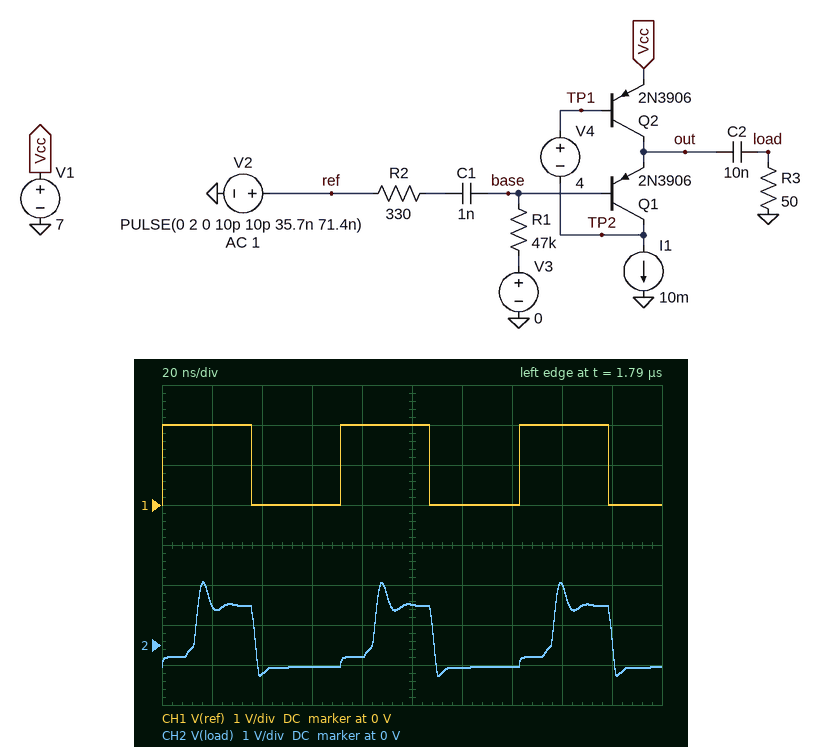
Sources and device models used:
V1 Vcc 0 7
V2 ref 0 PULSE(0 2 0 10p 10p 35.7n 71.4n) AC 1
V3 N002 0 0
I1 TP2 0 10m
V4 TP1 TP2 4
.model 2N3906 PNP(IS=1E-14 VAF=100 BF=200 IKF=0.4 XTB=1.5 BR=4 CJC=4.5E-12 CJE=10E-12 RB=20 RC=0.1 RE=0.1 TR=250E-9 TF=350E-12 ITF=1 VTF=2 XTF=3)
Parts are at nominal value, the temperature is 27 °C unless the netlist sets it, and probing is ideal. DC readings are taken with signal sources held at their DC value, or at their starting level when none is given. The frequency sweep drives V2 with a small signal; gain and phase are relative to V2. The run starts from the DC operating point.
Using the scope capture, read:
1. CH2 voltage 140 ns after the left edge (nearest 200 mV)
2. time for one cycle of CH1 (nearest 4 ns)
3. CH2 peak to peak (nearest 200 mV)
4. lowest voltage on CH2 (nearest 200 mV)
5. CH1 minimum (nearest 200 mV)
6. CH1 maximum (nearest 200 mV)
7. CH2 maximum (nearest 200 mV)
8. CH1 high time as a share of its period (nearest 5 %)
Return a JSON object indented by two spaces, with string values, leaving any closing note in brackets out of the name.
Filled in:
{
  "CH2 voltage 140 ns after the left edge": "-600 mV",
  "time for one cycle of CH1": "72 ns",
  "CH2 peak to peak": "2.4 V",
  "lowest voltage on CH2": "-800 mV",
  "CH1 minimum": "0 V",
  "CH1 maximum": "2.0 V",
  "CH2 maximum": "1.6 V",
  "CH1 high time as a share of its period": "50 %"
}
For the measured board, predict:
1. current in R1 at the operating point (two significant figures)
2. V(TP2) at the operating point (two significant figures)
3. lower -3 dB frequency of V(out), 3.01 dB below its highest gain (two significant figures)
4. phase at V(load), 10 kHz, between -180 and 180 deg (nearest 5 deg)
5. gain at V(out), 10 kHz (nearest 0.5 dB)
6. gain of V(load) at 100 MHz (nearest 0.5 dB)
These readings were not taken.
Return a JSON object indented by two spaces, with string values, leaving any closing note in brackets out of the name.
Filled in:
{
  "current in R1 at the operating point": "51 µA",
  "V(TP2) at the operating point": "2.3 V",
  "lower -3 dB frequency of V(out), 3.01 dB below its highest gain": "3.9 kHz",
  "phase at V(load), 10 kHz, between -180 and 180 deg": "105 deg",
  "gain at V(out), 10 kHz": "-0.5 dB",
  "gain of V(load) at 100 MHz": "-2.0 dB"
}
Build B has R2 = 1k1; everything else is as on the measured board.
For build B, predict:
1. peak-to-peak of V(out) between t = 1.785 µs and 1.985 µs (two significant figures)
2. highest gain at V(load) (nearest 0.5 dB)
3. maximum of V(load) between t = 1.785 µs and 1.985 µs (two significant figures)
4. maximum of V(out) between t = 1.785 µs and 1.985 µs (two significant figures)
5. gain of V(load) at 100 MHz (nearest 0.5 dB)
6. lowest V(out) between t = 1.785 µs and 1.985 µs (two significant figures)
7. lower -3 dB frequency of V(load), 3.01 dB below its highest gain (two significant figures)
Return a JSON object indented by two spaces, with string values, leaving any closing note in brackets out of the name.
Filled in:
{
  "peak-to-peak of V(out) between t = 1.785 µs and 1.985 µs": "1.7 V",
  "highest gain at V(load)": "-0.5 dB",
  "maximum of V(load) between t = 1.785 µs and 1.985 µs": "1.1 V",
  "maximum of V(out) between t = 1.785 µs and 1.985 µs": "5.1 V",
  "gain of V(load) at 100 MHz": "-13.0 dB",
  "lowest V(out) between t = 1.785 µs and 1.985 µs": "3.5 V",
  "lower -3 dB frequency of V(load), 3.01 dB below its highest gain": "310 kHz"
}
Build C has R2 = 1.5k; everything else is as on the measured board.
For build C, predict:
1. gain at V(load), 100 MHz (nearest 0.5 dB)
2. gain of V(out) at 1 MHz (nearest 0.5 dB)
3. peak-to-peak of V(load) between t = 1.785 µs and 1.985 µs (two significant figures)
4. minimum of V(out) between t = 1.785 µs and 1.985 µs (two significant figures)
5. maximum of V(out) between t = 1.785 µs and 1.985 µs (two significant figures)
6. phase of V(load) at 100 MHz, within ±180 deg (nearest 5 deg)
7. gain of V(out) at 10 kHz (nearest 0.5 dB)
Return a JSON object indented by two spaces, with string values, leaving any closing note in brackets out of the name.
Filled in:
{
  "gain at V(load), 100 MHz": "-16.0 dB",
  "gain of V(out) at 1 MHz": "-0.5 dB",
  "peak-to-peak of V(load) between t = 1.785 µs and 1.985 µs": "1.6 V",
  "minimum of V(out) between t = 1.785 µs and 1.985 µs": "3.5 V",
  "maximum of V(out) between t = 1.785 µs and 1.985 µs": "5.0 V",
  "phase of V(load) at 100 MHz, within ±180 deg": "-120 deg",
  "gain of V(out) at 10 kHz": "-1.0 dB"
}
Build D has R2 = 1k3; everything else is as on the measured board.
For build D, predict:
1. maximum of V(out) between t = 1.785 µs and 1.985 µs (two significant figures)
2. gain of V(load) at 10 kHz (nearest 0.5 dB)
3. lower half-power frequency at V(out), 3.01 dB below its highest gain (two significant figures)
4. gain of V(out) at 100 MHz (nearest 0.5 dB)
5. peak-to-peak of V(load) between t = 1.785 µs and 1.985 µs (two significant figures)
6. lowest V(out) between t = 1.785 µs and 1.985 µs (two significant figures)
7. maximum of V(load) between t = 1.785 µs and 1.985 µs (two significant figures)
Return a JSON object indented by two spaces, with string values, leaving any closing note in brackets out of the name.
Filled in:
{
  "maximum of V(out) between t = 1.785 µs and 1.985 µs": "5.1 V",
  "gain of V(load) at 10 kHz": "-31.0 dB",
  "lower half-power frequency at V(out), 3.01 dB below its highest gain": "3.4 kHz",
  "gain of V(out) at 100 MHz": "-14.5 dB",
  "peak-to-peak of V(load) between t = 1.785 µs and 1.985 µs": "1.6 V",
  "lowest V(out) between t = 1.785 µs and 1.985 µs": "3.5 V",
  "maximum of V(load) between t = 1.785 µs and 1.985 µs": "1.1 V"
}
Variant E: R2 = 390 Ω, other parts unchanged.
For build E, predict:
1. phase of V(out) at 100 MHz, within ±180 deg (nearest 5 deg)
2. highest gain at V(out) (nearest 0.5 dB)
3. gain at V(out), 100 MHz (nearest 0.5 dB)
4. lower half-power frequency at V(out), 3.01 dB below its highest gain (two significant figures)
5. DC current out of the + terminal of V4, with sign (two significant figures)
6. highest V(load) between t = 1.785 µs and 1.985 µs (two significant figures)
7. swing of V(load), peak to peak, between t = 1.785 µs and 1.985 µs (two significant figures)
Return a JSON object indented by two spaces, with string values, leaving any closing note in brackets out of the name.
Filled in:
{
  "phase of V(out) at 100 MHz, within ±180 deg": "-95 deg",
  "highest gain at V(out)": "0 dB",
  "gain at V(out), 100 MHz": "-3.5 dB",
  "lower half-power frequency at V(out), 3.01 dB below its highest gain": "3.7 kHz",
  "DC current out of the + terminal of V4, with sign": "-50 µA",
  "highest V(load) between t = 1.785 µs and 1.985 µs": "1.5 V",
  "swing of V(load), peak to peak, between t = 1.785 µs and 1.985 µs": "2.2 V"
}
